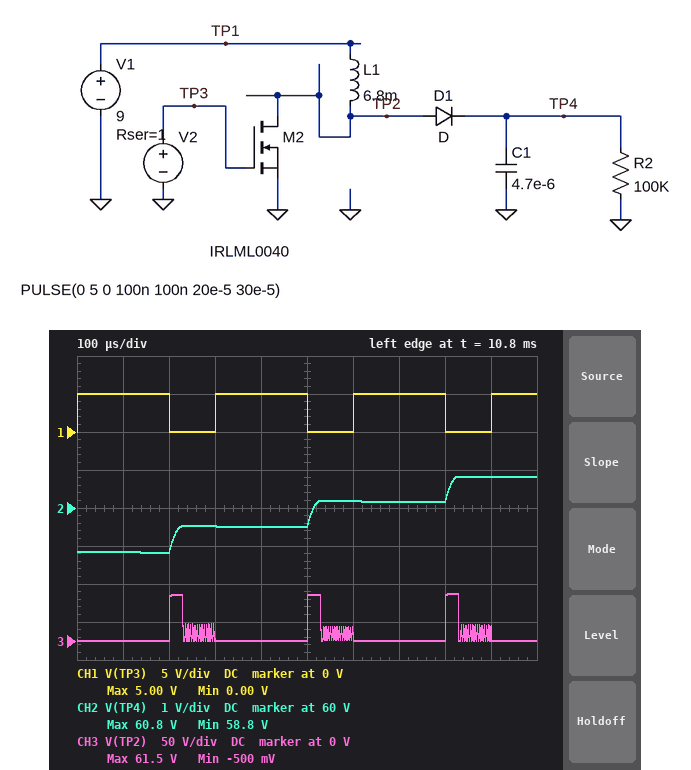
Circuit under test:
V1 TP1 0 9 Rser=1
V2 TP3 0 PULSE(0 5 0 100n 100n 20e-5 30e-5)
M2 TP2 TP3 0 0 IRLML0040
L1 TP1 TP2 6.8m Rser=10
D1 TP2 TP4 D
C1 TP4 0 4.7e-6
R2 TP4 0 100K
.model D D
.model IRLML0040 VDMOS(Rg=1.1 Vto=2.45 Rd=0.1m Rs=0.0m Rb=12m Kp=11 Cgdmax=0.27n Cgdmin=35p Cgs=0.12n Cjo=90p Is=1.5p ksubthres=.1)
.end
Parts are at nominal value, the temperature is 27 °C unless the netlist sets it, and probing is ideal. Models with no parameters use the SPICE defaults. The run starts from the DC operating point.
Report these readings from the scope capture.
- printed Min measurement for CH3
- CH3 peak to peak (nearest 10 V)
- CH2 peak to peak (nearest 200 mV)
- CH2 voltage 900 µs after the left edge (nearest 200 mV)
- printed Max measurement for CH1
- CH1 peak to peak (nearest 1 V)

-500 mV
60 V
2.0 V
60.8 V
5.00 V
5 V
